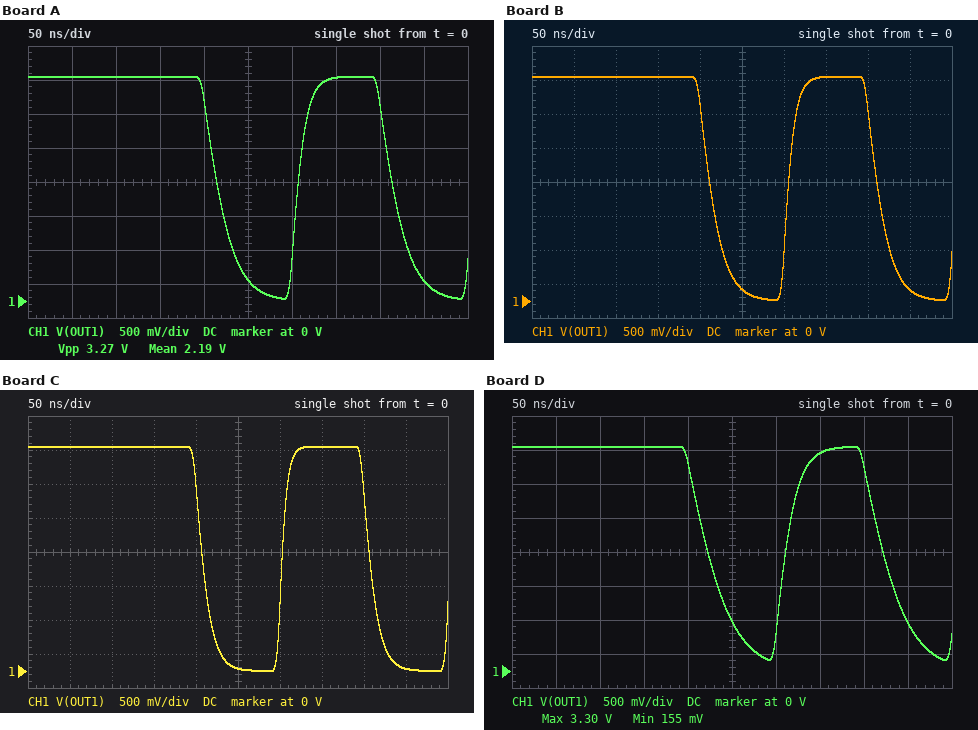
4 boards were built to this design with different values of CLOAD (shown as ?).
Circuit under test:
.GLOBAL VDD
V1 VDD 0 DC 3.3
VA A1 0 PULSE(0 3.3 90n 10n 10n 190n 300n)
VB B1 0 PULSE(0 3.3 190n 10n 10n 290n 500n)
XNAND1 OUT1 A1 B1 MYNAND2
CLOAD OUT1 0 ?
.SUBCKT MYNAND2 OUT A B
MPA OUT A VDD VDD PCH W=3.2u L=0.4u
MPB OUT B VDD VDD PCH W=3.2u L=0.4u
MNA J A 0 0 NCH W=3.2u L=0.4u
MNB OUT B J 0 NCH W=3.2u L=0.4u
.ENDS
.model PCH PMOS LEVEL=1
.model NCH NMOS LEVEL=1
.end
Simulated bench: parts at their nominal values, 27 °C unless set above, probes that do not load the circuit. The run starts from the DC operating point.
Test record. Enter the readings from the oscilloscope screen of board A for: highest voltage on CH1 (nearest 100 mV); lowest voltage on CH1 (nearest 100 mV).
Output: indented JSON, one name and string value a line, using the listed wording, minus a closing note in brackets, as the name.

{
  "highest voltage on CH1": "3.3 V",
  "lowest voltage on CH1": "0 V"
}
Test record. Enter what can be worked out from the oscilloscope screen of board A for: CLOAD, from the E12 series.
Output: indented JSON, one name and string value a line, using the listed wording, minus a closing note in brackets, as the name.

{
  "CLOAD, from the E12 series": "4.7 pF"
}
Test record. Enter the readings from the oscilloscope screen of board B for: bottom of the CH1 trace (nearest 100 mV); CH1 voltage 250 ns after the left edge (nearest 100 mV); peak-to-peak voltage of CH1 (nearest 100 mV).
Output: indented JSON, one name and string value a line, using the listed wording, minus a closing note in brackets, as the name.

{
  "bottom of the CH1 trace": "0 V",
  "CH1 voltage 250 ns after the left edge": "200 mV",
  "peak-to-peak voltage of CH1": "3.3 V"
}
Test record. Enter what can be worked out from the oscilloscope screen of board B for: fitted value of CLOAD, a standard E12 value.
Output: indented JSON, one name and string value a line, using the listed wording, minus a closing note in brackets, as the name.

{
  "fitted value of CLOAD, a standard E12 value": "3.9 pF"
}
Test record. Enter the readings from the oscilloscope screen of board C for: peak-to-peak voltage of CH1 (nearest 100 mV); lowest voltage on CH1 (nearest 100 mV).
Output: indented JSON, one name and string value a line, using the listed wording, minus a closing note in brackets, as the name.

{
  "peak-to-peak voltage of CH1": "3.3 V",
  "lowest voltage on CH1": "0 V"
}
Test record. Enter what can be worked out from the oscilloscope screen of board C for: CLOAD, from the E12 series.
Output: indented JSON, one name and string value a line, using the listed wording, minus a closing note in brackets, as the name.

{
  "CLOAD, from the E12 series": "2.7 pF"
}
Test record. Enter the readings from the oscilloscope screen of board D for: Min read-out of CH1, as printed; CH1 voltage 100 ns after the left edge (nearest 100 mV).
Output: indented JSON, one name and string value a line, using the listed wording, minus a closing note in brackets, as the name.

{
  "Min read-out of CH1, as printed": "155 mV",
  "CH1 voltage 100 ns after the left edge": "3.3 V"
}
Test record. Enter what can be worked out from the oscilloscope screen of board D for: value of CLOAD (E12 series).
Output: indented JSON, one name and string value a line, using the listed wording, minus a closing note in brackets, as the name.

{
  "value of CLOAD": "6.8 pF"
}
